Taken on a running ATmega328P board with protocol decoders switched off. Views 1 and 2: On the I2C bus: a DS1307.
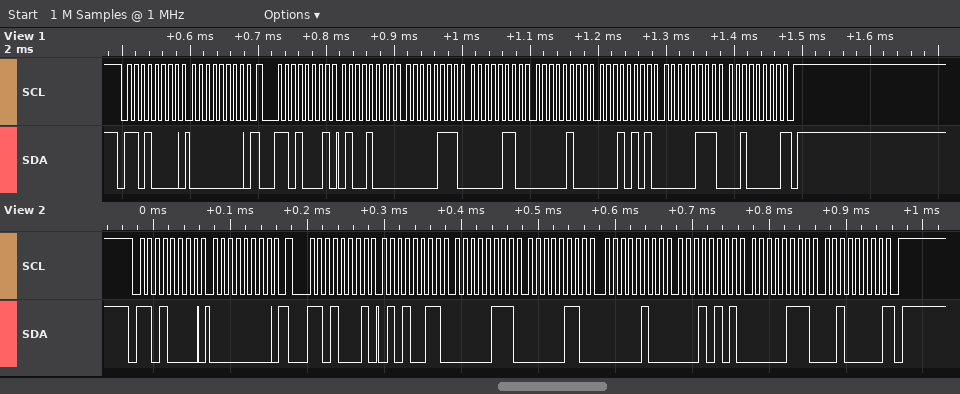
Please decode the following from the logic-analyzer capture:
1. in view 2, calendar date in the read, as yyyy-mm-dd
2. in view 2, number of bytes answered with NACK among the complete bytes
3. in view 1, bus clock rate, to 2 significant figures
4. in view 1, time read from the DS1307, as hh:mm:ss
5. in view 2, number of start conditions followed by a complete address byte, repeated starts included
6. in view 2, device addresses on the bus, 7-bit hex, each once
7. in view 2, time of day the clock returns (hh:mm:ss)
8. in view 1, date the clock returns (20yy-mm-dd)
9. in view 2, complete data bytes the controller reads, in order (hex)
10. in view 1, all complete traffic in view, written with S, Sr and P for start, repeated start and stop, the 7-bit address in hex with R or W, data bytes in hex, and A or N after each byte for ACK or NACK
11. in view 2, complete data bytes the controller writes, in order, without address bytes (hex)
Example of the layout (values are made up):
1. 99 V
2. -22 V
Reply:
1. 2020-07-15
2. 1
3. 100 kHz
4. 06:07:48
5. 2
6. 0x68
7. 06:07:53
8. 2020-07-15
9. 53 07 06 04 15 07 20
10. S 68W A 00 A Sr 68R A 48 A 07 A 06 A 04 A 15 A 07 A 20 N P
11. 00
